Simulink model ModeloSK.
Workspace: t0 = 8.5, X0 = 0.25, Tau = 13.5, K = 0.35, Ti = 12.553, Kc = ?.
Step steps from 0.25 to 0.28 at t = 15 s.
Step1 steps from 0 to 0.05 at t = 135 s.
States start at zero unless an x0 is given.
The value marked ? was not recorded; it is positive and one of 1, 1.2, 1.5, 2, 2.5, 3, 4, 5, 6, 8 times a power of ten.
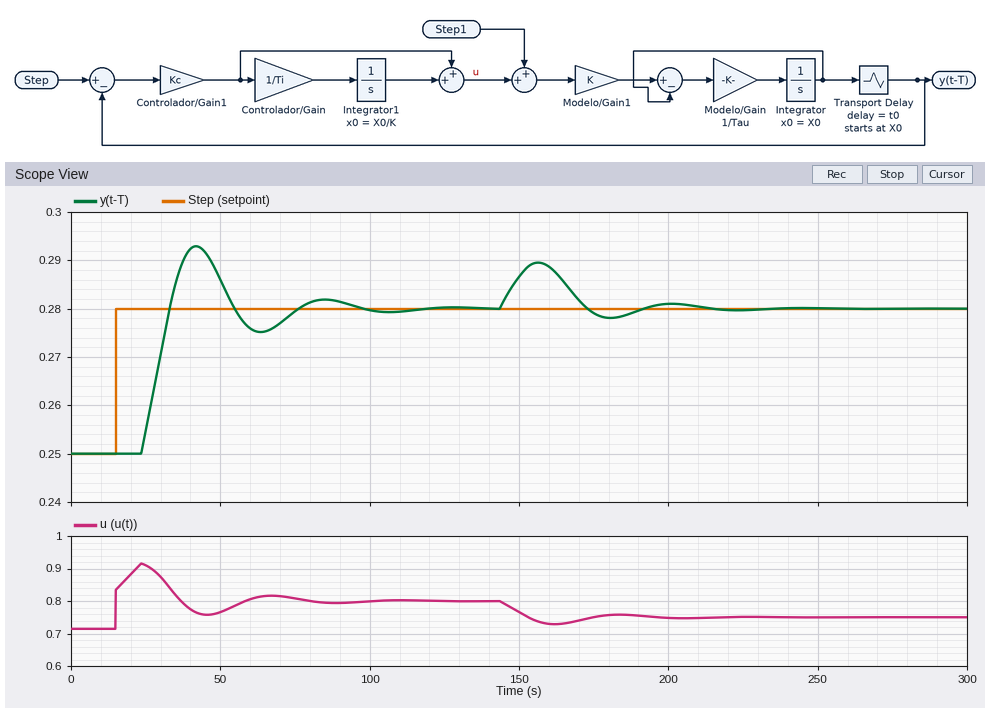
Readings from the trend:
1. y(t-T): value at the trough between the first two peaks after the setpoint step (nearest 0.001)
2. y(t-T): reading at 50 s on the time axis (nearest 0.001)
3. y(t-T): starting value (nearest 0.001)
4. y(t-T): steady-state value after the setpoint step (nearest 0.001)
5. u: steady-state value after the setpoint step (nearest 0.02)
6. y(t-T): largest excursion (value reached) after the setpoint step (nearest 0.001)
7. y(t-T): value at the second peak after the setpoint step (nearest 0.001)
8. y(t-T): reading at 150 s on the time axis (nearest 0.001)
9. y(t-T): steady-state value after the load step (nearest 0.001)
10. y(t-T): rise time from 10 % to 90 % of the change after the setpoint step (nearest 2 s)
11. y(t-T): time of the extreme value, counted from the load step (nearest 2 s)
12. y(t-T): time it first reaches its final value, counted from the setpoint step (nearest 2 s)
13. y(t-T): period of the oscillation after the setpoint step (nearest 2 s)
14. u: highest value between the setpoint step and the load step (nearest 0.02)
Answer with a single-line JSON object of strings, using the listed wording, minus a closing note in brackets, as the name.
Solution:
{"y(t-T): value at the trough between the first two peaks after the setpoint step": "0.275", "y(t-T): reading at 50 s on the time axis": "0.286", "y(t-T): starting value": "0.250", "y(t-T): steady-state value after the setpoint step": "0.280", "u: steady-state value after the setpoint step": "0.80", "y(t-T): largest excursion (value reached) after the setpoint step": "0.293", "y(t-T): value at the second peak after the setpoint step": "0.282", "y(t-T): reading at 150 s on the time axis": "0.287", "y(t-T): steady-state value after the load step": "0.280", "y(t-T): rise time from 10 % to 90 % of the change after the setpoint step": "8 s", "y(t-T): time of the extreme value, counted from the load step": "22 s", "y(t-T): time it first reaches its final value, counted from the setpoint step": "18 s", "y(t-T): period of the oscillation after the setpoint step": "44 s", "u: highest value between the setpoint step and the load step": "0.92"}
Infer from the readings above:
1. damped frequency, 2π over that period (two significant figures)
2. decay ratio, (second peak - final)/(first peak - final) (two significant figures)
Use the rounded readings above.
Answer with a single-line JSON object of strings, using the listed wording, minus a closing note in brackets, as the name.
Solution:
{"damped frequency, 2π over that period": "0.14 rad/s", "decay ratio, (second peak - final)/(first peak - final)": "0.15"}
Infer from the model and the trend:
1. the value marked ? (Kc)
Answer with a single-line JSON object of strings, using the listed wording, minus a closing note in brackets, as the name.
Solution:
{"the value marked ?": "4"}
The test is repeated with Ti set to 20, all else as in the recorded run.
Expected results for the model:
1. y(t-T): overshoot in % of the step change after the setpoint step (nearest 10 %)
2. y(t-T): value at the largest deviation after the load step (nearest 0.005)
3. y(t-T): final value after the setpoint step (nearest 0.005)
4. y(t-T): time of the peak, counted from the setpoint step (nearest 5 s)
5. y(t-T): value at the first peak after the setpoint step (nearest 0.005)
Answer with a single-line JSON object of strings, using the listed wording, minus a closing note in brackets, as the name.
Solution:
{"y(t-T): overshoot in % of the step change after the setpoint step": "20 %", "y(t-T): value at the largest deviation after the load step": "0.290", "y(t-T): final value after the setpoint step": "0.280", "y(t-T): time of the peak, counted from the setpoint step": "25 s", "y(t-T): value at the first peak after the setpoint step": "0.285"}
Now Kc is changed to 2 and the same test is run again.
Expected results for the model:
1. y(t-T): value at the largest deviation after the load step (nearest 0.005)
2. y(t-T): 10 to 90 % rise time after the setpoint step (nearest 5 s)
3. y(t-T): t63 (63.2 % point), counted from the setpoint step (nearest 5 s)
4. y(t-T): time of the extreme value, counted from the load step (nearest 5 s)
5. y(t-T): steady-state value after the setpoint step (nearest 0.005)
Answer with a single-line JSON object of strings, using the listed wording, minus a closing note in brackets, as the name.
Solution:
{"y(t-T): value at the largest deviation after the load step": "0.290", "y(t-T): 10 to 90 % rise time after the setpoint step": "20 s", "y(t-T): t63 (63.2 % point), counted from the setpoint step": "20 s", "y(t-T): time of the extreme value, counted from the load step": "25 s", "y(t-T): steady-state value after the setpoint step": "0.280"}
